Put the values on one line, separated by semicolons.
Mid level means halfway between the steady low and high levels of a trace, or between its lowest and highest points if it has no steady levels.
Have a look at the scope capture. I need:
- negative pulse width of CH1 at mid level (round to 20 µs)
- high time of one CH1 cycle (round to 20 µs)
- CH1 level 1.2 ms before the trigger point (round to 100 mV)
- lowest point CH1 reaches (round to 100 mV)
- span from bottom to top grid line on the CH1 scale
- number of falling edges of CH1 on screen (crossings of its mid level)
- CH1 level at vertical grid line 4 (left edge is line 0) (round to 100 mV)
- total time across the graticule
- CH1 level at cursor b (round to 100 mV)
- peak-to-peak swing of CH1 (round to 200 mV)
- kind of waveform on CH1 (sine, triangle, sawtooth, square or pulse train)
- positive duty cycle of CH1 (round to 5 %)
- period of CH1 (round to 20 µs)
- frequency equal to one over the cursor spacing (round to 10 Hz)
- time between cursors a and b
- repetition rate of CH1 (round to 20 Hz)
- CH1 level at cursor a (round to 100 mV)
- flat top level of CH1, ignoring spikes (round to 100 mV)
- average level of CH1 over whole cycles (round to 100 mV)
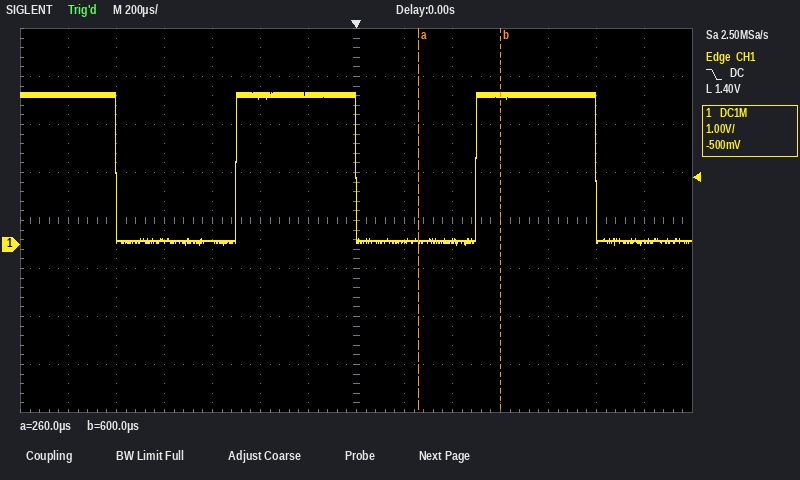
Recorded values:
500 µs; 500 µs; 3.1 V; 0.0 V; 8 V; 3; 100 mV; 2.8 ms; 3.1 V; 3.2 V; square; 50 %; 1.00 ms; 2.94 kHz; 340 µs; 1.00 kHz; 100 mV; 3.1 V; 1.6 V
